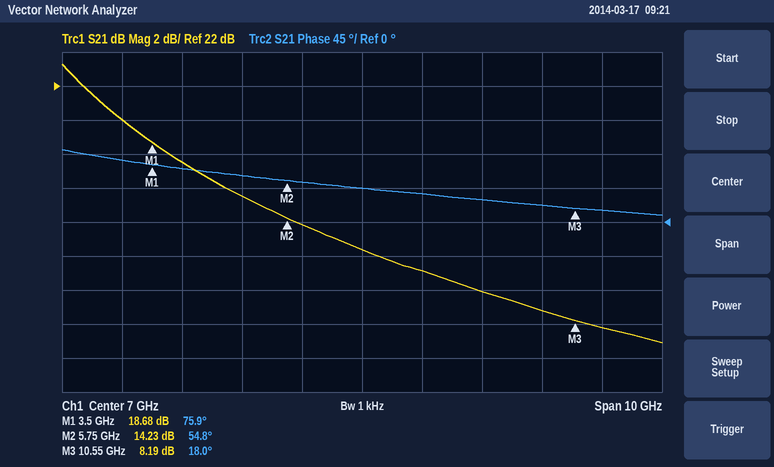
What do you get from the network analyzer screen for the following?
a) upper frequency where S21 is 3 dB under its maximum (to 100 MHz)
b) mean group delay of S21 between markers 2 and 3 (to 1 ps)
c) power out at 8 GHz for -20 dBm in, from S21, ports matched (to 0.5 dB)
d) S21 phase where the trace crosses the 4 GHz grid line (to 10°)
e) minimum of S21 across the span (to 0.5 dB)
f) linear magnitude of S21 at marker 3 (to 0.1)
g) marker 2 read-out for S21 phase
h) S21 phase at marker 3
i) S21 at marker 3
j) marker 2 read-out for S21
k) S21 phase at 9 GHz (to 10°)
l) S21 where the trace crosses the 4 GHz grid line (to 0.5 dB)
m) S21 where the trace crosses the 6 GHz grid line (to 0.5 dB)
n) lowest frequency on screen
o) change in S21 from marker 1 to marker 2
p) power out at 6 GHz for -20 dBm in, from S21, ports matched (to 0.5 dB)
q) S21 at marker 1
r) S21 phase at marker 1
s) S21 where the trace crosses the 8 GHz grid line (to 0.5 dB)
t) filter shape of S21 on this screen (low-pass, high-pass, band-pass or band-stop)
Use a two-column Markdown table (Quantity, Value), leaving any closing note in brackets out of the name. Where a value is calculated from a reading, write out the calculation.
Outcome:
| Quantity | Value |
|---|---|
| upper frequency where S21 is 3 dB under its maximum | 2.9 GHz |
| mean group delay of S21 between markers 2 and 3 | −(18° − (54.8°))/(360° × 4.8 GHz) ≈ 21 ps |
| power out at 8 GHz for -20 dBm in, from S21, ports matched | -20 dBm + (11.0 dB) = -9.0 dBm |
| S21 phase where the trace crosses the 4 GHz grid line | 70° |
| minimum of S21 across the span | 7.0 dB |
| linear magnitude of S21 at marker 3 | 10^(8.19/20) ≈ 2.6 |
| marker 2 read-out for S21 phase | 54.8° |
| S21 phase at marker 3 | 18.0° |
| S21 at marker 3 | 8.19 dB |
| marker 2 read-out for S21 | 14.23 dB |
| S21 phase at 9 GHz | 30° |
| S21 where the trace crosses the 4 GHz grid line | 17.5 dB |
| S21 where the trace crosses the 6 GHz grid line | 14.0 dB |
| lowest frequency on screen | 2 GHz |
| change in S21 from marker 1 to marker 2 | 14.23 − (18.68) = -4.45 dB |
| power out at 6 GHz for -20 dBm in, from S21, ports matched | -20 dBm + (14.0 dB) = -6.0 dBm |
| S21 at marker 1 | 18.68 dB |
| S21 phase at marker 1 | 75.9° |
| S21 where the trace crosses the 8 GHz grid line | 11.0 dB |
| filter shape of S21 on this screen | low-pass |
